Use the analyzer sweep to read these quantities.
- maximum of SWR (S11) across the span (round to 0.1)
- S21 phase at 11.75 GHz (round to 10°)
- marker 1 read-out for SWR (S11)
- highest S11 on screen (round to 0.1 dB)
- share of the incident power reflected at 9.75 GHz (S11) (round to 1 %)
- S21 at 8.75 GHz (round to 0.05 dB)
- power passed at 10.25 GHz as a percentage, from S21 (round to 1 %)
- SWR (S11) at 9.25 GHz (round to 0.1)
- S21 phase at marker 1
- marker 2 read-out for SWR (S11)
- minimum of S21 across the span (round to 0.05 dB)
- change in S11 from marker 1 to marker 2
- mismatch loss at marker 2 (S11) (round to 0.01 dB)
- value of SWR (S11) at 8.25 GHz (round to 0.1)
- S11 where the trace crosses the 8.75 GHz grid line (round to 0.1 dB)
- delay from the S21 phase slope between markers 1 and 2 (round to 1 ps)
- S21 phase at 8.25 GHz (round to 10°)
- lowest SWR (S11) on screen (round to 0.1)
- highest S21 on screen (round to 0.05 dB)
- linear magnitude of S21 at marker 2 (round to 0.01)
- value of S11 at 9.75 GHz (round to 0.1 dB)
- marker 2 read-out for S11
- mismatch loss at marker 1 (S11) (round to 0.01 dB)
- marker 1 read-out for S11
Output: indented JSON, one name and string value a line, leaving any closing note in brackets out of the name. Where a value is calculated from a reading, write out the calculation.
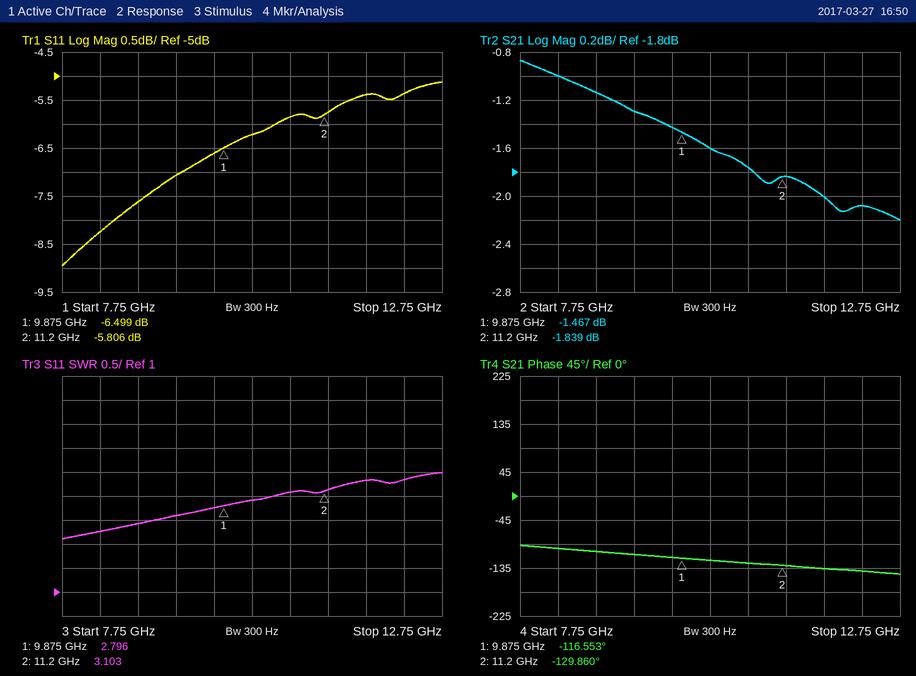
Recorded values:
{
  "maximum of SWR (S11) across the span": "3.5",
  "S21 phase at 11.75 GHz": "-140°",
  "marker 1 read-out for SWR": "2.796",
  "highest S11 on screen": "-5.1 dB",
  "share of the incident power reflected at 9.75 GHz (S11)": "10^(-6.6/10) ≈ 22 %",
  "S21 at 8.75 GHz": "-1.15 dB",
  "power passed at 10.25 GHz as a percentage, from S21": "10^(-1.6/10) ≈ 69 %",
  "SWR (S11) at 9.25 GHz": "2.6",
  "S21 phase at marker 1": "-116.553°",
  "marker 2 read-out for SWR": "3.103",
  "minimum of S21 across the span": "-2.20 dB",
  "change in S11 from marker 1 to marker 2": "-5.806 − (-6.499) = 0.693 dB",
  "mismatch loss at marker 2 (S11)": "−10 log10(1 − 10^(-5.806/10)) ≈ 1.32 dB",
  "value of SWR (S11) at 8.25 GHz": "2.3",
  "S11 where the trace crosses the 8.75 GHz grid line": "-7.6 dB",
  "delay from the S21 phase slope between markers 1 and 2": "−(-129.86° − (-116.553°))/(360° × 1.325 GHz) ≈ 28 ps",
  "S21 phase at 8.25 GHz": "-100°",
  "lowest SWR (S11) on screen": "2.1",
  "highest S21 on screen": "-0.85 dB",
  "linear magnitude of S21 at marker 2": "10^(-1.839/20) ≈ 0.81",
  "value of S11 at 9.75 GHz": "-6.6 dB",
  "marker 2 read-out for S11": "-5.806 dB",
  "mismatch loss at marker 1 (S11)": "−10 log10(1 − 10^(-6.499/10)) ≈ 1.10 dB",
  "marker 1 read-out for S11": "-6.499 dB"
}
